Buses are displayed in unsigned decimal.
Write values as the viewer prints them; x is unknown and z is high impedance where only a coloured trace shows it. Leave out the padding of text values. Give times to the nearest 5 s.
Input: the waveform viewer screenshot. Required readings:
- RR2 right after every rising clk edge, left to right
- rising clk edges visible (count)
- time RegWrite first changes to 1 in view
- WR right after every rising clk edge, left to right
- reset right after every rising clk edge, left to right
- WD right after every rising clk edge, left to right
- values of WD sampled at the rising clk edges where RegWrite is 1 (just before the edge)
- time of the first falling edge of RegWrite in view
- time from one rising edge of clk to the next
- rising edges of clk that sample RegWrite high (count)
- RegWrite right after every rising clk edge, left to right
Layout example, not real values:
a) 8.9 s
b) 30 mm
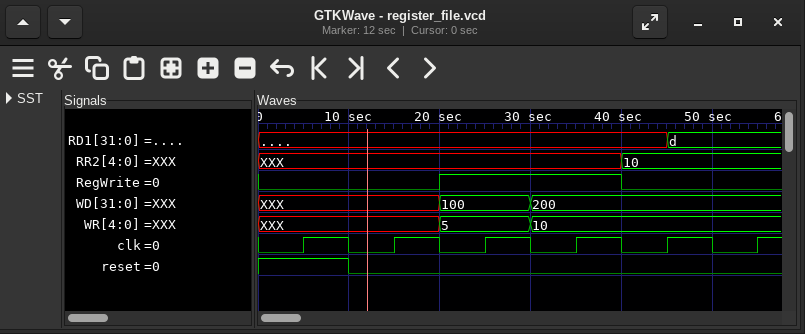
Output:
a) XXX, XXX, XXX, XXX, 10, 10
b) 6
c) 20 s
d) XXX, XXX, 5, 10, 10, 10
e) 1 0 0 0 0 0
f) XXX, XXX, 100, 200, 200, 200
g) 100, 200
h) 40 s
i) 10 s
j) 2
k) 0 0 1 1 0 0
